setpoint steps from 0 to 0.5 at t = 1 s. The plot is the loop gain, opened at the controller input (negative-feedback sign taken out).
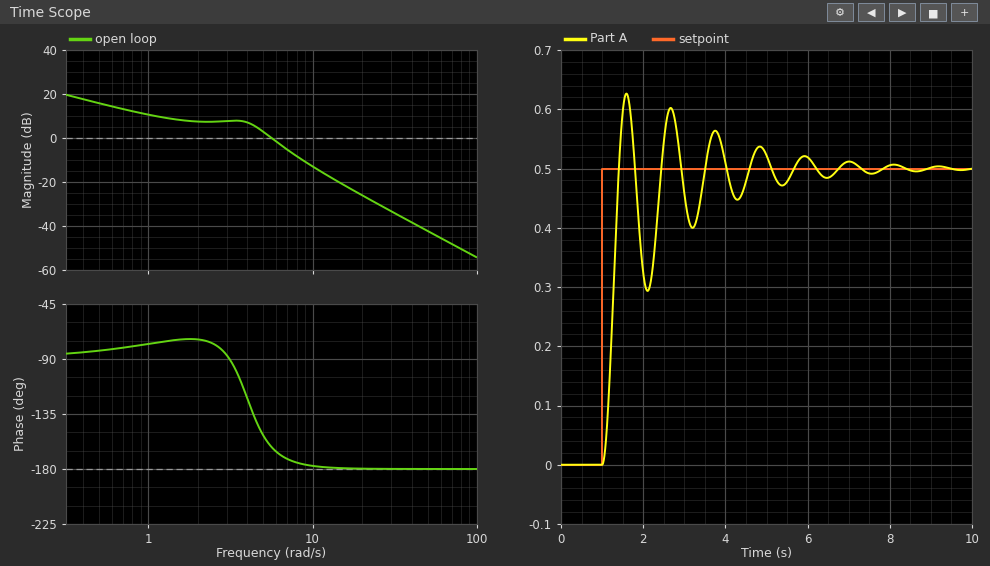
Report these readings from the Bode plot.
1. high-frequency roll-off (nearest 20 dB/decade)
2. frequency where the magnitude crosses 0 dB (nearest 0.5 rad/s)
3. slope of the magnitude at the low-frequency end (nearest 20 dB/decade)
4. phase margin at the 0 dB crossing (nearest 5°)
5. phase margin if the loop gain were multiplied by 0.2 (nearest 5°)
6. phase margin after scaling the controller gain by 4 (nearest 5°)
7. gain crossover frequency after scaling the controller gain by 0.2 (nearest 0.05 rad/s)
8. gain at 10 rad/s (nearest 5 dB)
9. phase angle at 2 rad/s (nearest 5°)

-40 dB/decade
5.5 rad/s
-20 dB/decade
20°
100°
5°
0.65 rad/s
-15 dB
-75°
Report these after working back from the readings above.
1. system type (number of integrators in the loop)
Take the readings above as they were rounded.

1
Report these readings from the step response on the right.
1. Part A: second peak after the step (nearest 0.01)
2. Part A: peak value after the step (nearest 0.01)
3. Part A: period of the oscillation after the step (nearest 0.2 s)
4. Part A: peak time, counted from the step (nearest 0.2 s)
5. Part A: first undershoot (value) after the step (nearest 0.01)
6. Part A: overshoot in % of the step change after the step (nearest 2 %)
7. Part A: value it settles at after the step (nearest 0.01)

0.60
0.63
1.0 s
0.6 s
0.29
26 %
0.50
